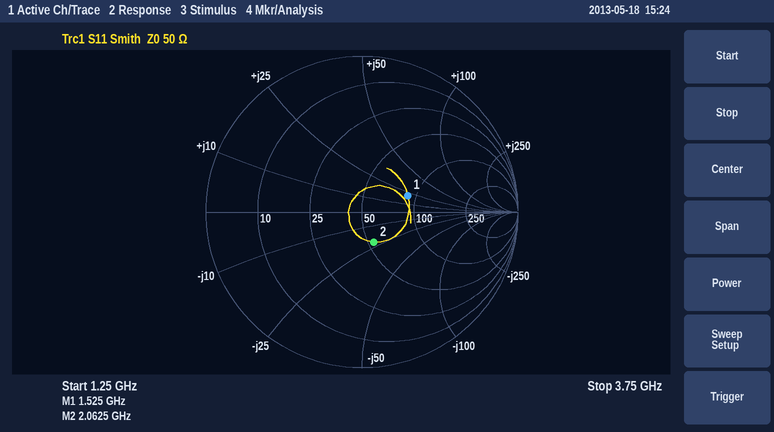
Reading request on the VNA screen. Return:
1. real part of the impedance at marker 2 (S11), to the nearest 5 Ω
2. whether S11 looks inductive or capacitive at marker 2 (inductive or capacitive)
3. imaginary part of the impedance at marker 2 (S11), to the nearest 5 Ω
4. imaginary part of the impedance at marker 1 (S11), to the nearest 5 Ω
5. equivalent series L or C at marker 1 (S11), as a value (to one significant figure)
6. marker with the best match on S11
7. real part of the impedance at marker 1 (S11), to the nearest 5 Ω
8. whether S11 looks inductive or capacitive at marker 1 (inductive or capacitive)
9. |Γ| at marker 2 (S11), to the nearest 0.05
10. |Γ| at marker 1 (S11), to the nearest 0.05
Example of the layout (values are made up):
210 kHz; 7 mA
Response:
55 Ω; capacitive; -20 Ω; +20 Ω; 2 nH; marker 2; 90 Ω; inductive; 0.20; 0.30
